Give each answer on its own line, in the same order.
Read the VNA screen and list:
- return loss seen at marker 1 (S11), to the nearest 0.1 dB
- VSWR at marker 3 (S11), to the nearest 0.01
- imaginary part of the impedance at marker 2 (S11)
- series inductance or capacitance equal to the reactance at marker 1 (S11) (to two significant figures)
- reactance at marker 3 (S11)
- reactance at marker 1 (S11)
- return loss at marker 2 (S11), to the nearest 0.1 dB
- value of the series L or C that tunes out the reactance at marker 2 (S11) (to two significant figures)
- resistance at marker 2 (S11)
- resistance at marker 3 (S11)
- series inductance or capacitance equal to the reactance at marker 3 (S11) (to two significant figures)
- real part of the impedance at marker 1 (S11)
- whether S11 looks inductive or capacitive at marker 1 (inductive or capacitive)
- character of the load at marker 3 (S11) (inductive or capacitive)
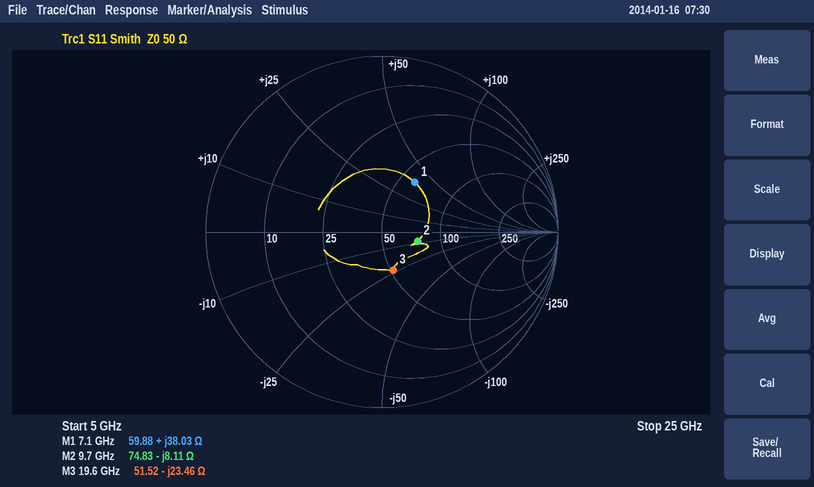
9.4 dB
1.58
-8.11 Ω
850 pH
-23.46 Ω
+38.03 Ω
13.6 dB
130 pH
74.83 Ω
51.52 Ω
350 fF
59.88 Ω
inductive
capacitive
